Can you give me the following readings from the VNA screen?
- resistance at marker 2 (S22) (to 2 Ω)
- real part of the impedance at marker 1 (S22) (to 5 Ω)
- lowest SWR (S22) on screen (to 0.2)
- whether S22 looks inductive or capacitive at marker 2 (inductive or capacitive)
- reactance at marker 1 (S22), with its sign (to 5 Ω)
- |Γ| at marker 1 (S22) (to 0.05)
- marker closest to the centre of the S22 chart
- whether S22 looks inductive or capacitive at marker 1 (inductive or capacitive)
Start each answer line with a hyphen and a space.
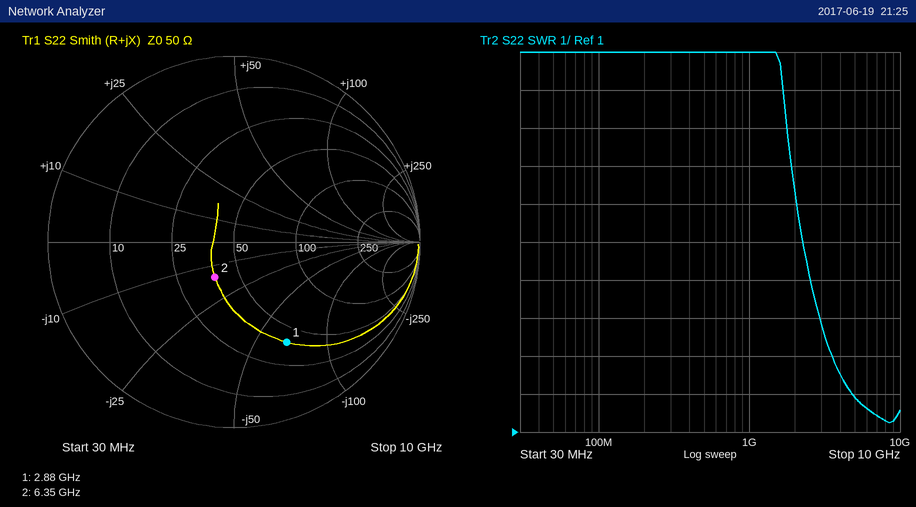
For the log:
- 38 Ω
- 40 Ω
- 1.2
- capacitive
- -65 Ω
- 0.60
- marker 2
- capacitive
